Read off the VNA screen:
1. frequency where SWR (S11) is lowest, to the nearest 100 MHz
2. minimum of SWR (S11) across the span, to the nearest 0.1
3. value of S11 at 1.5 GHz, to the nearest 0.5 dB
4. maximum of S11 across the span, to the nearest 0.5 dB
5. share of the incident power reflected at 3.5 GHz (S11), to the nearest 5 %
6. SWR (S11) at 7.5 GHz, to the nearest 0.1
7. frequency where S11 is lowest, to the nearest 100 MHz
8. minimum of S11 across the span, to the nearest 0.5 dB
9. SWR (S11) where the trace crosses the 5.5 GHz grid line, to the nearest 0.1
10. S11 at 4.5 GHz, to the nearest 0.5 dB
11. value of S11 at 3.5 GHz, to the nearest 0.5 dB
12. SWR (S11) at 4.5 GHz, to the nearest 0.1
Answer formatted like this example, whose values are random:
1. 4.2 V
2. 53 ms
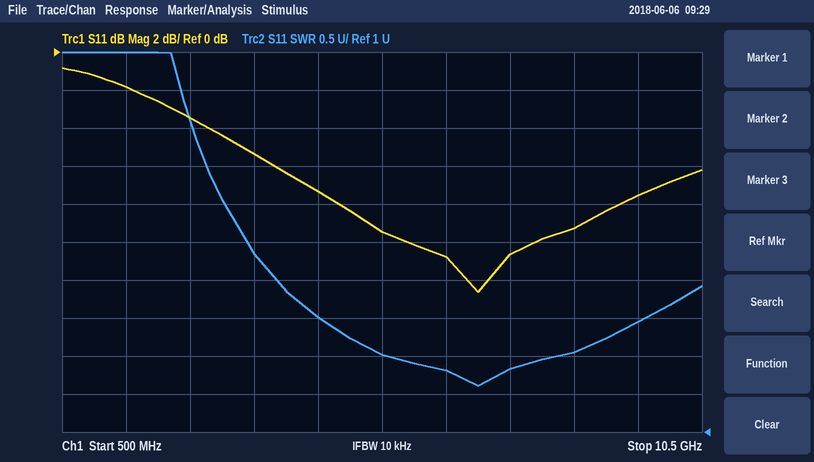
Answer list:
1. 7.0 GHz
2. 1.6
3. -2.0 dB
4. -1.0 dB
5. 30 %
6. 1.8
7. 7.0 GHz
8. -12.5 dB
9. 2.0
10. -7.5 dB
11. -5.5 dB
12. 2.5
